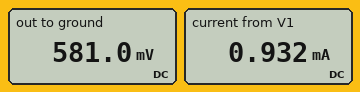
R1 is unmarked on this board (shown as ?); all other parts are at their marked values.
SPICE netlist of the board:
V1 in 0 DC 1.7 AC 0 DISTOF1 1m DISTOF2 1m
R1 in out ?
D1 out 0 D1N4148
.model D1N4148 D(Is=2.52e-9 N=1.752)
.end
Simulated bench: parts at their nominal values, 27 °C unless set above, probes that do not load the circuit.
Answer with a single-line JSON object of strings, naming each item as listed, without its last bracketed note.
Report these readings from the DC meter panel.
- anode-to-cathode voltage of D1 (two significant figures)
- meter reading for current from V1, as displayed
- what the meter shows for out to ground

{"anode-to-cathode voltage of D1": "580 mV", "meter reading for current from V1, as displayed": "0.932 mA", "what the meter shows for out to ground": "581.0 mV"}
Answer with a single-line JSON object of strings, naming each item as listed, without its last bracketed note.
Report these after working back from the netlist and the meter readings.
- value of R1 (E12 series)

{"value of R1": "1.2 kΩ"}
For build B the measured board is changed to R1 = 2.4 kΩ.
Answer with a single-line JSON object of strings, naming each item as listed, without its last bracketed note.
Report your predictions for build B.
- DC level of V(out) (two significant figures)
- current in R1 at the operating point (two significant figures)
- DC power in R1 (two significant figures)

{"DC level of V(out)": "550 mV", "current in R1 at the operating point": "480 µA", "DC power in R1": "550 µW"}
